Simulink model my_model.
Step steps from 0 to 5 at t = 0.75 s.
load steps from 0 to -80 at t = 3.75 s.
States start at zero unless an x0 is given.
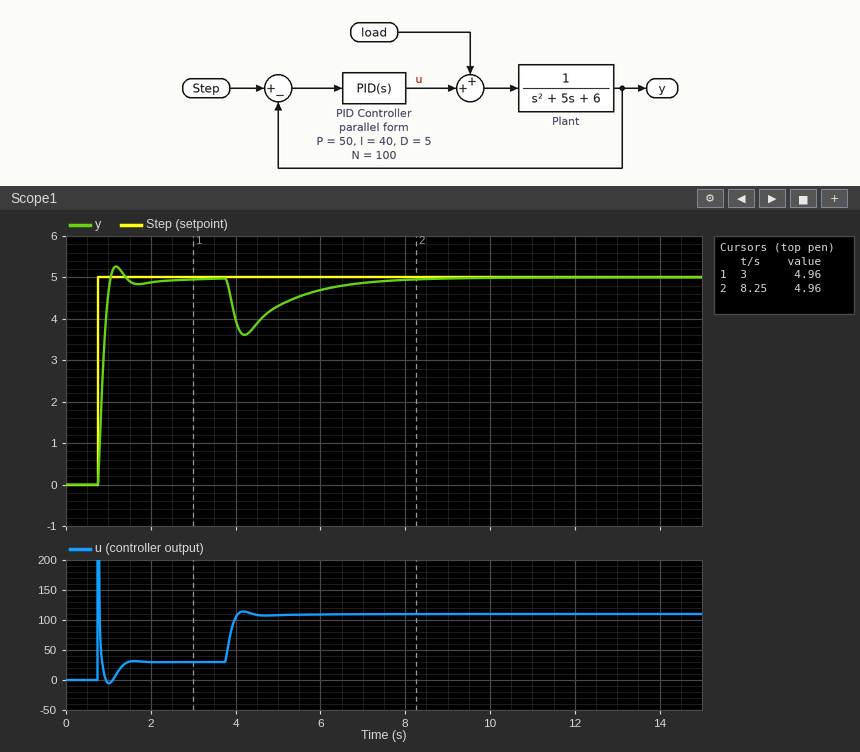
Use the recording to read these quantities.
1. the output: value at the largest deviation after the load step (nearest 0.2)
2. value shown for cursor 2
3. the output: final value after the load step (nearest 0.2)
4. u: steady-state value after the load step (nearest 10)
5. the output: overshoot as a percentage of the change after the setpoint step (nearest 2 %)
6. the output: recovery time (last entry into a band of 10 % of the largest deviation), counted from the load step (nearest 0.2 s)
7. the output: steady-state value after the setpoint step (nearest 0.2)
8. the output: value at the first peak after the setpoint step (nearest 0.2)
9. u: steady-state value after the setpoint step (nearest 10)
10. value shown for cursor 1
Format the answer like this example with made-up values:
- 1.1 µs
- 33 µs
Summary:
- 3.6
- 4.96
- 5.0
- 110
- 6 %
- 3.2 s
- 5.0
- 5.2
- 30
- 4.96
